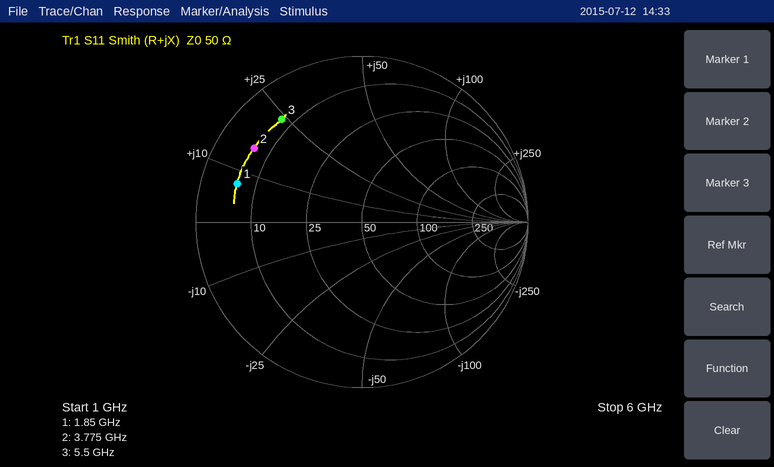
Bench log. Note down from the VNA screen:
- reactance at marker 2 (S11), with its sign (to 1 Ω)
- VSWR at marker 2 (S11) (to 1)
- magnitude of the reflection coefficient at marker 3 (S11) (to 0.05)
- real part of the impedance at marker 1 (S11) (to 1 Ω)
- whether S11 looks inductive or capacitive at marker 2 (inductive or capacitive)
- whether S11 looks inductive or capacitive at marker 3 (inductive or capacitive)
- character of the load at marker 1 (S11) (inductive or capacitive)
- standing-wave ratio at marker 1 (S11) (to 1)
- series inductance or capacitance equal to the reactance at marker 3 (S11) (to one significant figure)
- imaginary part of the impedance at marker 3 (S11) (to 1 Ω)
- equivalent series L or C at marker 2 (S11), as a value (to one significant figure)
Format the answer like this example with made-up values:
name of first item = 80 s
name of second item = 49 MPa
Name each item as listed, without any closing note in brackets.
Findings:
reactance at marker 2 (S11), with its sign = +15 Ω
VSWR at marker 2 (S11) = 8
magnitude of the reflection coefficient at marker 3 (S11) = 0.80
real part of the impedance at marker 1 (S11) = 6 Ω
whether S11 looks inductive or capacitive at marker 2 = inductive
whether S11 looks inductive or capacitive at marker 3 = inductive
character of the load at marker 1 (S11) = inductive
standing-wave ratio at marker 1 (S11) = 8
series inductance or capacitance equal to the reactance at marker 3 (S11) = 700 pH
imaginary part of the impedance at marker 3 (S11) = +24 Ω
equivalent series L or C at marker 2 (S11), as a value = 600 pH
